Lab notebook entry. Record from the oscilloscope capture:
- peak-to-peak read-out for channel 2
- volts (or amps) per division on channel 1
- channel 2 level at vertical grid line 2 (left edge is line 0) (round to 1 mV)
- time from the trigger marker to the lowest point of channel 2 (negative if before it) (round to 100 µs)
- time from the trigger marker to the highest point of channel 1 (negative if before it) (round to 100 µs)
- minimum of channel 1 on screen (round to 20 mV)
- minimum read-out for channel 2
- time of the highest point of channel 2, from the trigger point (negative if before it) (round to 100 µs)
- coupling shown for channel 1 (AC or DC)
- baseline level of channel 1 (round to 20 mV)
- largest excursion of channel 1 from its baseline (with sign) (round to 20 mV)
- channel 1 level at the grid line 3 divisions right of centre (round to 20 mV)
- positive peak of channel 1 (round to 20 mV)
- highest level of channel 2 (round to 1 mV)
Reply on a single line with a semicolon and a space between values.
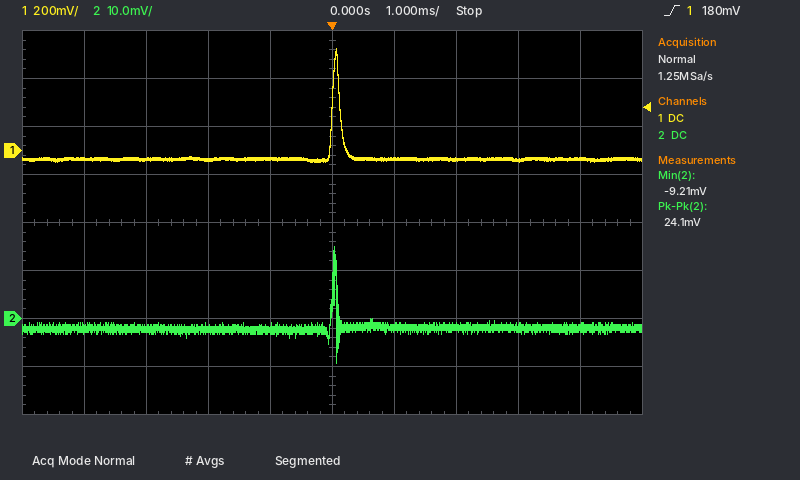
24.1 mV; 200 mV; -2 mV; +100 µs; +100 µs; -40 mV; -9.21 mV; 0.0 ms; DC; -40 mV; +460 mV; -40 mV; 420 mV; 15 mV
